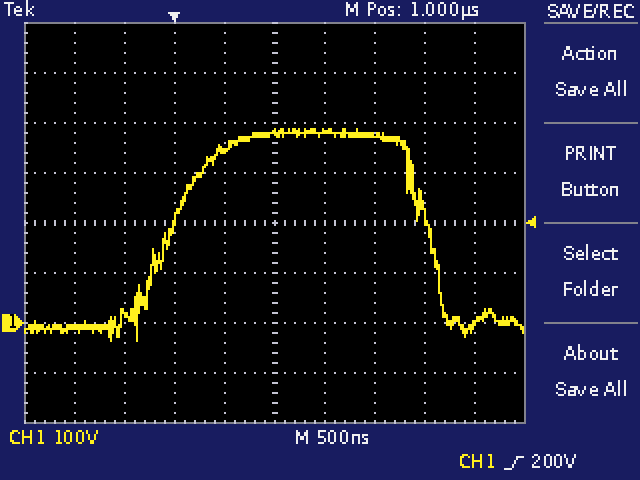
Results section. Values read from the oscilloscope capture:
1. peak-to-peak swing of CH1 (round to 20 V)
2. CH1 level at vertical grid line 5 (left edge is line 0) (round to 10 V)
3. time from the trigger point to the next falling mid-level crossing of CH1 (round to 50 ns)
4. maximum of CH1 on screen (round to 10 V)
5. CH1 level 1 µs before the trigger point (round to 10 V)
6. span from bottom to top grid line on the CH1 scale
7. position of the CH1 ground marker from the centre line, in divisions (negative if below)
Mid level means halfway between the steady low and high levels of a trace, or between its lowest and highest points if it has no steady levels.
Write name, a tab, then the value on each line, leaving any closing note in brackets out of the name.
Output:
peak-to-peak swing of CH1	420 V
CH1 level at vertical grid line 5 (left edge is line 0)	380 V
time from the trigger point to the next falling mid-level crossing of CH1	2.55 µs
maximum of CH1 on screen	390 V
CH1 level 1 µs before the trigger point	-10 V
span from bottom to top grid line on the CH1 scale	800 V
position of the CH1 ground marker from the centre line, in divisions	-2.0 div
